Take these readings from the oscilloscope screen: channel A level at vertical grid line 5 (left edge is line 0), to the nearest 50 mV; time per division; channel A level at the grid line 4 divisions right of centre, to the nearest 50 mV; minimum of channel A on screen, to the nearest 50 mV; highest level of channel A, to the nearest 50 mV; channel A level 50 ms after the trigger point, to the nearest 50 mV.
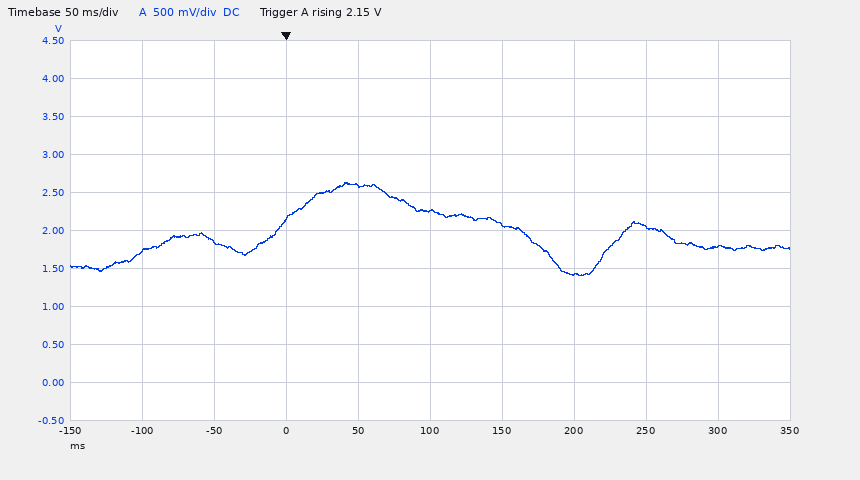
2.25 V
50 ms
1.80 V
1.40 V
2.65 V
2.60 V
